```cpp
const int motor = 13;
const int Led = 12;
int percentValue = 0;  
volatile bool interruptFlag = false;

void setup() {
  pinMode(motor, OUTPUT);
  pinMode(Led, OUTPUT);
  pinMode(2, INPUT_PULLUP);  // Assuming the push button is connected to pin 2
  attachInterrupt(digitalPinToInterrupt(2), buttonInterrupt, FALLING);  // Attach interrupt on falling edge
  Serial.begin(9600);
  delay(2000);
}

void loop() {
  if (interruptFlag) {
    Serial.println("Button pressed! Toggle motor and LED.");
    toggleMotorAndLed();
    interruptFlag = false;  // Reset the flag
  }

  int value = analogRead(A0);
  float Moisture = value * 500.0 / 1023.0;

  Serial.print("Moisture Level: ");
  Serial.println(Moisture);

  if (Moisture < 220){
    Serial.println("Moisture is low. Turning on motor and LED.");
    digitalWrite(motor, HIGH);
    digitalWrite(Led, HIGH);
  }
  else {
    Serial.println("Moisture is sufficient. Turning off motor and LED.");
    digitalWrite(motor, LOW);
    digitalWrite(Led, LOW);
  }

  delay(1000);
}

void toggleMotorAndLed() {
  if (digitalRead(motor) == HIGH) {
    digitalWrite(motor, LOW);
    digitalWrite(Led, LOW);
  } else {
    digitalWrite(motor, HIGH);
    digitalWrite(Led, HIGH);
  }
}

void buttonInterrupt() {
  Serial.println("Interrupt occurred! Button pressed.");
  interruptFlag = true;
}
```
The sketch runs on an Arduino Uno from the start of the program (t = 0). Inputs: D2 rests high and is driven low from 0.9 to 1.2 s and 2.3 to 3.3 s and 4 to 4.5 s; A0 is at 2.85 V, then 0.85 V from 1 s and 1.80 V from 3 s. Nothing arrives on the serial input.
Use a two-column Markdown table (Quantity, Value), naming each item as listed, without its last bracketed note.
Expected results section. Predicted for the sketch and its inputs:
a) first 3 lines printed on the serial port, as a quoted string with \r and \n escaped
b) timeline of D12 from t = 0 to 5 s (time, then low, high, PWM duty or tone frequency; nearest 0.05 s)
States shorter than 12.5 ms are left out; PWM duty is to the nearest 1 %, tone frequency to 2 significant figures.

| Quantity | Value |
|---|---|
| first 3 lines printed on the serial port, as a quoted string with \r and \n escaped | "Interrupt occurred! Button pressed.\r\nButton pressed! Toggle motor and LED.\r\nMoisture Level: 85.04\r\n" |
| timeline of D12 from t = 0 to 5 s | 0 s low; 2 s high; 3.05 s low; 3.1 s high; 4.1 s low; 4.15 s high |
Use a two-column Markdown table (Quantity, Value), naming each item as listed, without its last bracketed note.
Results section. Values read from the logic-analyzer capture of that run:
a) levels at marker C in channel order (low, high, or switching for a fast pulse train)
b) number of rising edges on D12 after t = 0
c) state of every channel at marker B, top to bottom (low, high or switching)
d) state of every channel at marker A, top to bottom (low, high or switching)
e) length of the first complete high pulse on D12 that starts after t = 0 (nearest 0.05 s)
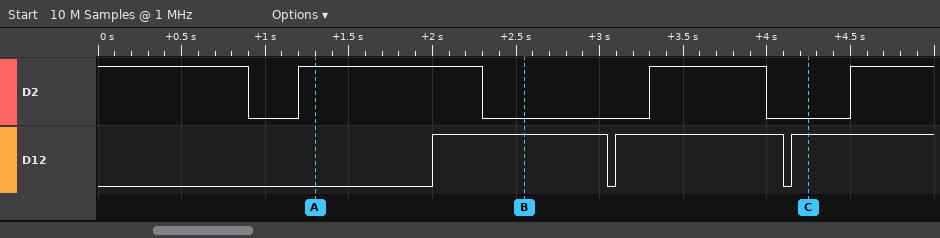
| Quantity | Value |
|---|---|
| levels at marker C in channel order | D2 low, D12 high |
| number of rising edges on D12 after t = 0 | 3 |
| state of every channel at marker B, top to bottom | D2 low, D12 high |
| state of every channel at marker A, top to bottom | D2 high, D12 low |
| length of the first complete high pulse on D12 that starts after t = 0 | 1.05 s |
